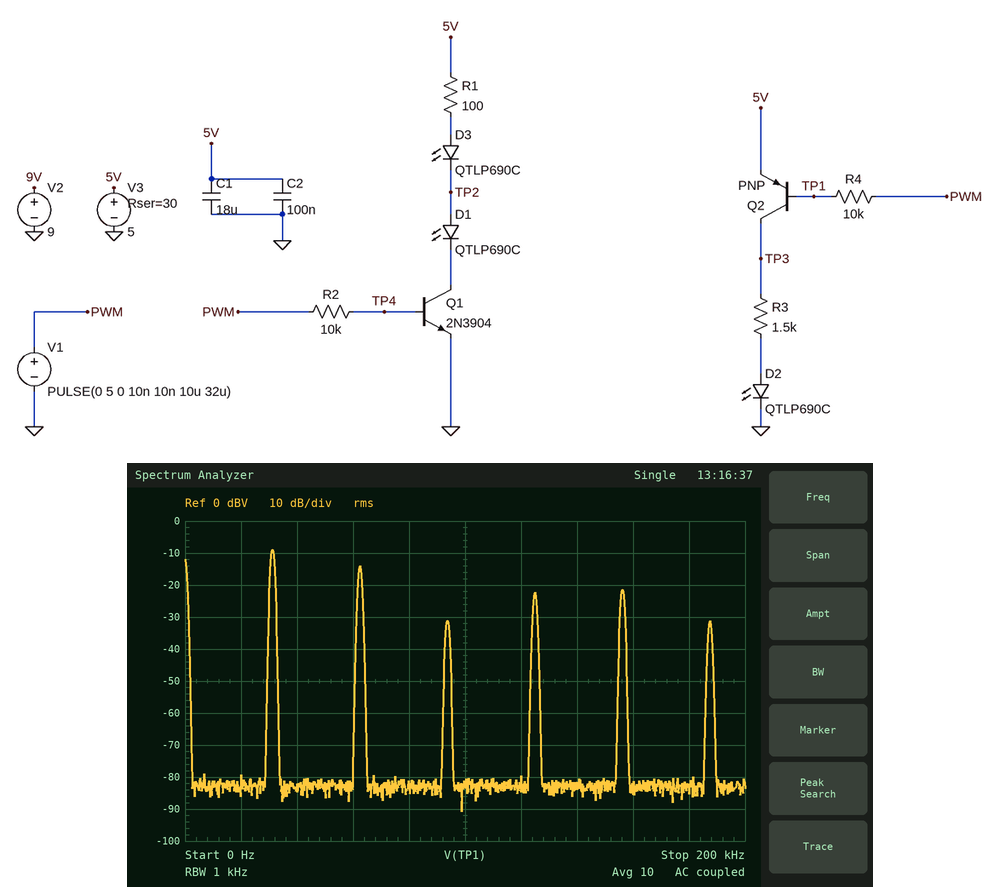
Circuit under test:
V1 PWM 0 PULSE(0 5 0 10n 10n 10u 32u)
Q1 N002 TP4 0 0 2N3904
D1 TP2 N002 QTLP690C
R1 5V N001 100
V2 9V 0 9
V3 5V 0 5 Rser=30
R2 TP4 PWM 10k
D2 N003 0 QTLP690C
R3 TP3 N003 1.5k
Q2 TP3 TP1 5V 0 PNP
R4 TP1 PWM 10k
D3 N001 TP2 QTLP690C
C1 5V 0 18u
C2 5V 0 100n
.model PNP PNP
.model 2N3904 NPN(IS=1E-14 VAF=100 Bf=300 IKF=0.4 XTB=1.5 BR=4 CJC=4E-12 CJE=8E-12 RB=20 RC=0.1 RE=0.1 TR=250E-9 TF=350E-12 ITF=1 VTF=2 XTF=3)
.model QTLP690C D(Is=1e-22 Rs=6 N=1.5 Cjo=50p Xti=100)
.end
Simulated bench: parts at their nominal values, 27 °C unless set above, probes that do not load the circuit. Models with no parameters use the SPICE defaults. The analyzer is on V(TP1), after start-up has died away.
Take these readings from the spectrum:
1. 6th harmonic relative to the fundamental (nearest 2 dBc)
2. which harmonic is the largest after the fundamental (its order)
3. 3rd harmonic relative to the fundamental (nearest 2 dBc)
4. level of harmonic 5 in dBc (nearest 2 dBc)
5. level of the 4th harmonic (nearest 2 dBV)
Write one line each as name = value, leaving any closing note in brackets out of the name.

6th harmonic relative to the fundamental = -22 dBc
which harmonic is the largest after the fundamental = 2
3rd harmonic relative to the fundamental = -22 dBc
level of harmonic 5 in dBc = -12 dBc
level of the 4th harmonic = -22 dBV
